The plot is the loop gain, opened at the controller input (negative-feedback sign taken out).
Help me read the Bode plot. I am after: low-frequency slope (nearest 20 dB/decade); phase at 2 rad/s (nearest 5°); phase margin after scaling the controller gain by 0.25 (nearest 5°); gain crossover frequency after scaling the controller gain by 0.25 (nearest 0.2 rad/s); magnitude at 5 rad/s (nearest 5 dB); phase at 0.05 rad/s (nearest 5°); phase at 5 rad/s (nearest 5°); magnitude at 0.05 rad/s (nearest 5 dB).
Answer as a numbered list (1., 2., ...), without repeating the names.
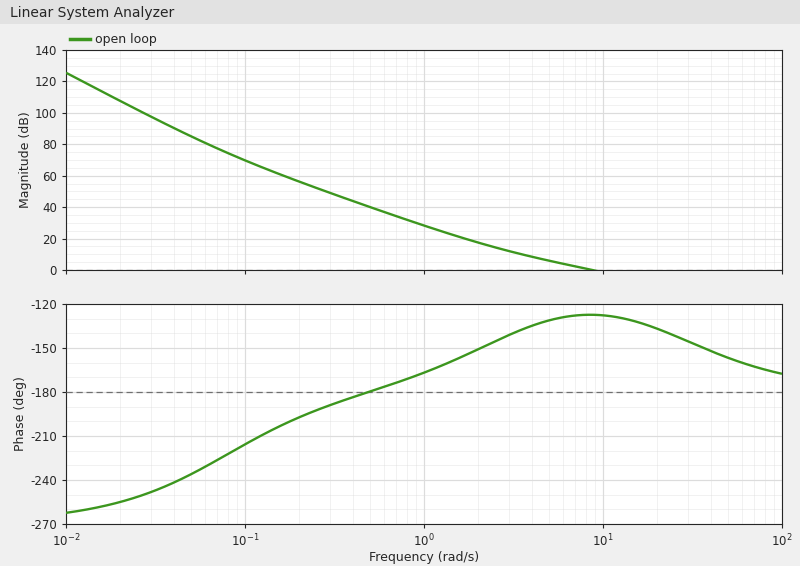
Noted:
1. -60 dB/decade
2. -150°
3. 40°
4. 3.0 rad/s
5. 5 dB
6. -235°
7. -130°
8. 85 dB
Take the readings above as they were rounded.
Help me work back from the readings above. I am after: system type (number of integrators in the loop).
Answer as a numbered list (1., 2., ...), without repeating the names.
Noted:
1. 3
